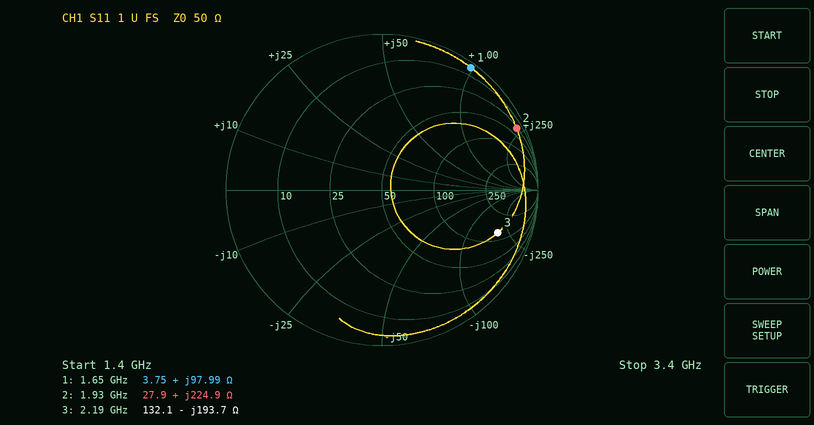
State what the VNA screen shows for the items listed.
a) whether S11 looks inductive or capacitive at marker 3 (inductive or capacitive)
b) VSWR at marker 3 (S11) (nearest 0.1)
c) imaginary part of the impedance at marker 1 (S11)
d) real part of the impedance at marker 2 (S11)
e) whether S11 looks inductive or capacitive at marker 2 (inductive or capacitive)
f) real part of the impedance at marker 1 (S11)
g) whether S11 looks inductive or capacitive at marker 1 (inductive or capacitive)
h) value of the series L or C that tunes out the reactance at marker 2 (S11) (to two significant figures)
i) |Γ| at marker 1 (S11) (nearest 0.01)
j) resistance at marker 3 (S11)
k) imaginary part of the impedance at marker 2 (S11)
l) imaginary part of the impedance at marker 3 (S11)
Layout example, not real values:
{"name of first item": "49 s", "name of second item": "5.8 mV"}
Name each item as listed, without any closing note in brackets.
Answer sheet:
{"whether S11 looks inductive or capacitive at marker 3": "capacitive", "VSWR at marker 3 (S11)": "8.6", "imaginary part of the impedance at marker 1": "+97.99 Ω", "real part of the impedance at marker 2": "27.9 Ω", "whether S11 looks inductive or capacitive at marker 2": "inductive", "real part of the impedance at marker 1": "3.75 Ω", "whether S11 looks inductive or capacitive at marker 1": "inductive", "value of the series L or C that tunes out the reactance at marker 2 (S11)": "370 fF", "|Γ| at marker 1 (S11)": "0.97", "resistance at marker 3": "132.1 Ω", "imaginary part of the impedance at marker 2": "+224.9 Ω", "imaginary part of the impedance at marker 3": "-193.7 Ω"}
